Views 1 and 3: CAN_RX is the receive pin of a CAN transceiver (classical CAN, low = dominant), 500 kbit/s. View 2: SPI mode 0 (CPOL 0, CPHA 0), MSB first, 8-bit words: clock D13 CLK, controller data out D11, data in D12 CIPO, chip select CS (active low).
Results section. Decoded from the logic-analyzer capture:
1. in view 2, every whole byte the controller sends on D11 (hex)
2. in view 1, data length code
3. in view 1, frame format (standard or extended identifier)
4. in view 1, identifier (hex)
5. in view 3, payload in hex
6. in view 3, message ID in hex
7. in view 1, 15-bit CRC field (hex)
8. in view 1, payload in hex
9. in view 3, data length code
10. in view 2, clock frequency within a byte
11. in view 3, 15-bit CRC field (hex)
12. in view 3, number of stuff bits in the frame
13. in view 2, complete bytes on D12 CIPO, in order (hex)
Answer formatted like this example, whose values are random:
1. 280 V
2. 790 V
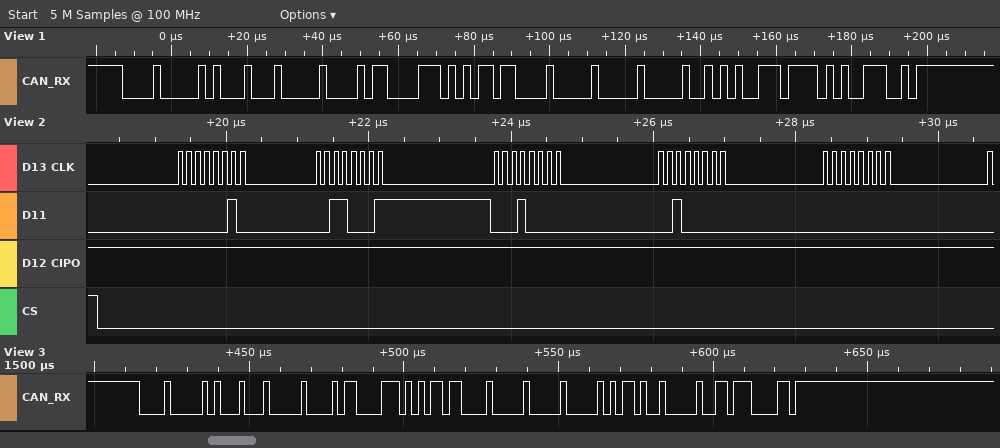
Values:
1. 0x02 0x31 0x10 0x20 0x00
2. 8
3. standard
4. 0x081
5. 80 2C 3A B6 10 00 0B 48
6. 0x081
7. 0x7A9C
8. 80 2C 3A B6 10 00 05 4E
9. 8
10. 8 MHz
11. 0x06E1
12. 6
13. 0xFF 0xFF 0xFF 0xFF 0xFF
